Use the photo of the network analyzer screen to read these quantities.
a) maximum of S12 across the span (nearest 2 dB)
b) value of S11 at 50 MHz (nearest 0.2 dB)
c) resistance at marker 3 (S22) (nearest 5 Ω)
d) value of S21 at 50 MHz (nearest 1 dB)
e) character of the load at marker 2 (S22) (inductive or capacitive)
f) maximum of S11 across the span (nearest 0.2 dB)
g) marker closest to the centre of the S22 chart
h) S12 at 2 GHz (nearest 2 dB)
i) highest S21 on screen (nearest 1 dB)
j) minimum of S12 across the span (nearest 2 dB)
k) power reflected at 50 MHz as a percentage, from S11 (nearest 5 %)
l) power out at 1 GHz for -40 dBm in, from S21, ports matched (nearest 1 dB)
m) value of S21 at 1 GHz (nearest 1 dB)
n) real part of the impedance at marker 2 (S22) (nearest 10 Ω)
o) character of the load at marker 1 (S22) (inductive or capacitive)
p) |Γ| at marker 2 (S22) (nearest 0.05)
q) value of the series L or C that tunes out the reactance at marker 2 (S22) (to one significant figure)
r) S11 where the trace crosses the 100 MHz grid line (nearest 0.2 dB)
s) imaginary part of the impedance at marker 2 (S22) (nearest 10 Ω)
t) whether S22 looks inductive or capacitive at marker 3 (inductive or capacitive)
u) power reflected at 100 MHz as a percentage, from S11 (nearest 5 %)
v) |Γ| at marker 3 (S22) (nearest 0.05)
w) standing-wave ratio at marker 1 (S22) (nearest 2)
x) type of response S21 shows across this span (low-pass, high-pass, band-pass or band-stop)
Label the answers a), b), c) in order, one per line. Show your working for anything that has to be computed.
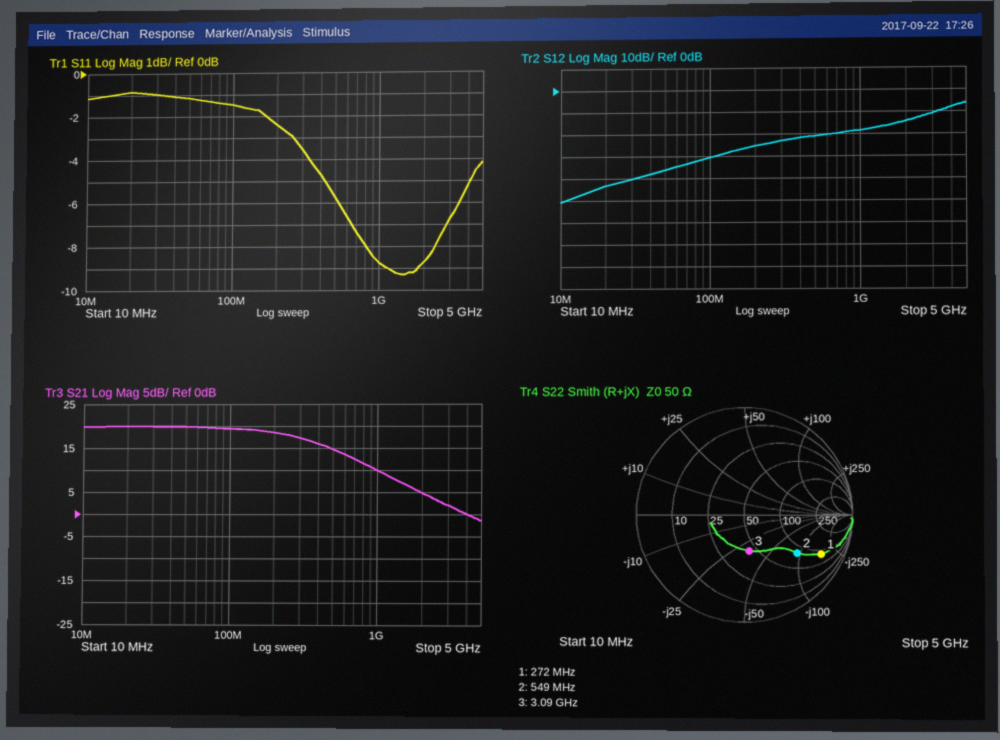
a) -6 dB
b) -1.2 dB
c) 45 Ω
d) 20 dB
e) capacitive
f) -0.8 dB
g) marker 3
h) -14 dB
i) 20 dB
j) -50 dB
k) 10^(-1.2/10) ≈ 75.9 %, so 75 % to the nearest 5 %
l) -40 dBm + (10 dB) = -30 dBm
m) 10 dB
n) 80 Ω
o) capacitive
p) 0.60
q) L = 90 Ω/(2π × 549 MHz) ≈ 26.1 nH, so 30 nH to one significant figure
r) -1.4 dB
s) -90 Ω
t) capacitive
u) 10^(-1.4/10) ≈ 72.4 %, so 70 % to the nearest 5 %
v) 0.35
w) 8
x) low-pass
